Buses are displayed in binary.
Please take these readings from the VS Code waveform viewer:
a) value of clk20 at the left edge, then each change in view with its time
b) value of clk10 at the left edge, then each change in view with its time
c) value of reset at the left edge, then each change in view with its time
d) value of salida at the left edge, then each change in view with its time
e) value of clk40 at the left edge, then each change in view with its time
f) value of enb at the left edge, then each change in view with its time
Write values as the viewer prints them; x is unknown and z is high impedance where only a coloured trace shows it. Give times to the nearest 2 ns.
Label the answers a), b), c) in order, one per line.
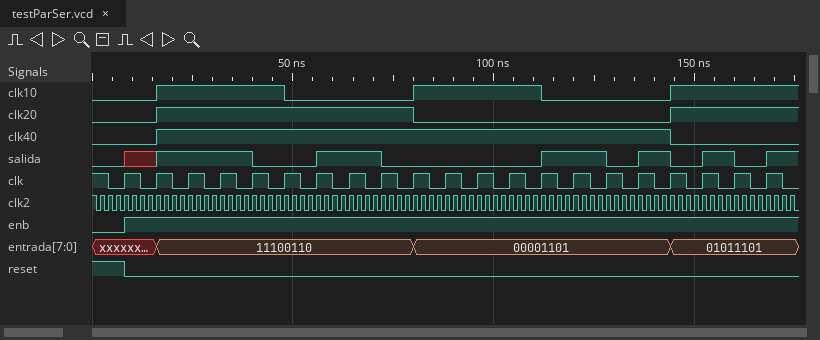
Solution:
a) 0, 1 at 16 ns, 0 at 80 ns, 1 at 144 ns
b) 0, 1 at 16 ns, 0 at 48 ns, 1 at 80 ns, 0 at 112 ns, 1 at 144 ns
c) 1, 0 at 8 ns
d) 0, x at 8 ns, 1 at 16 ns, 0 at 40 ns, 1 at 56 ns, 0 at 72 ns, 1 at 112 ns, 0 at 128 ns, 1 at 136 ns, 0 at 144 ns, 1 at 152 ns, 0 at 160 ns, 1 at 168 ns
e) 0, 1 at 16 ns, 0 at 144 ns
f) 0, 1 at 8 ns
